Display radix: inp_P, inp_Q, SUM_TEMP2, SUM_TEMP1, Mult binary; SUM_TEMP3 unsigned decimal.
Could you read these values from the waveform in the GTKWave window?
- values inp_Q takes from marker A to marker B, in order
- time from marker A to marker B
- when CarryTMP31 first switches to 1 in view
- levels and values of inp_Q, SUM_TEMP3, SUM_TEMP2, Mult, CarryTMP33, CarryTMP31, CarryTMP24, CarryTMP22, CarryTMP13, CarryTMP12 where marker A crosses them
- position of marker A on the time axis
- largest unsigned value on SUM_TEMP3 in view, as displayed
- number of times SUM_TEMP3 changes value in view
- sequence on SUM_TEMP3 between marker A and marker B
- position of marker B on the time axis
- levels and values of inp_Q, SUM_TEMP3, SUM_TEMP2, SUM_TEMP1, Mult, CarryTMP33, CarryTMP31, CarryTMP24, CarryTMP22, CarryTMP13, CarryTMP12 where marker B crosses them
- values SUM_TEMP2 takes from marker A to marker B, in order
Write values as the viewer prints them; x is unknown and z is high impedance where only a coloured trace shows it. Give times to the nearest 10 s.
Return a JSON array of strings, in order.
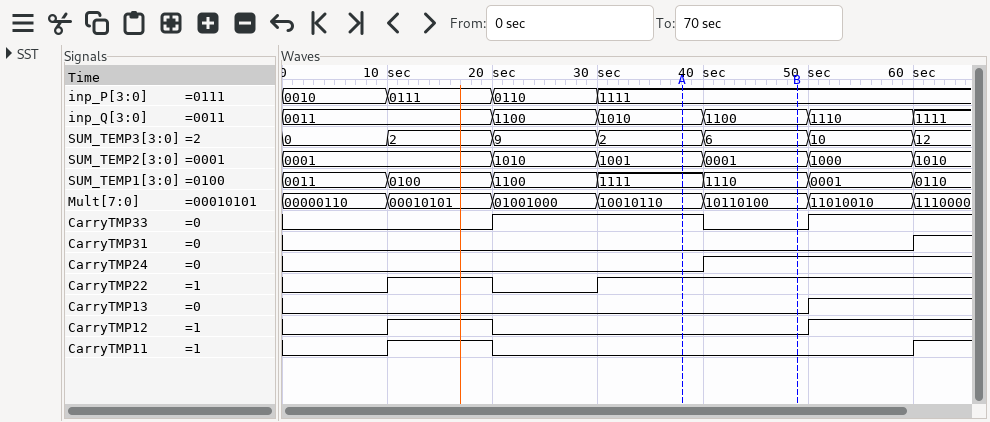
["1010, 1100", "10 s", "60 s", "inp_Q=1010, SUM_TEMP3=2, SUM_TEMP2=1001, Mult=10010110, CarryTMP33=1, CarryTMP31=0, CarryTMP24=0, CarryTMP22=1, CarryTMP13=0, CarryTMP12=0", "40 s", "12", "6", "2, 6", "50 s", "inp_Q=1100, SUM_TEMP3=6, SUM_TEMP2=0001, SUM_TEMP1=1110, Mult=10110100, CarryTMP33=0, CarryTMP31=0, CarryTMP24=1, CarryTMP22=1, CarryTMP13=0, CarryTMP12=0", "1001, 0001"]
